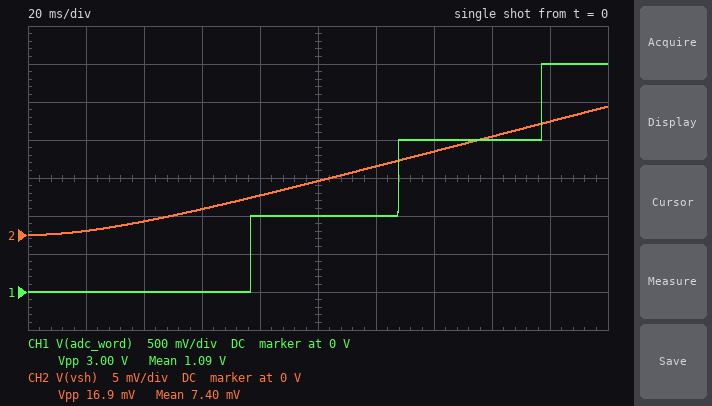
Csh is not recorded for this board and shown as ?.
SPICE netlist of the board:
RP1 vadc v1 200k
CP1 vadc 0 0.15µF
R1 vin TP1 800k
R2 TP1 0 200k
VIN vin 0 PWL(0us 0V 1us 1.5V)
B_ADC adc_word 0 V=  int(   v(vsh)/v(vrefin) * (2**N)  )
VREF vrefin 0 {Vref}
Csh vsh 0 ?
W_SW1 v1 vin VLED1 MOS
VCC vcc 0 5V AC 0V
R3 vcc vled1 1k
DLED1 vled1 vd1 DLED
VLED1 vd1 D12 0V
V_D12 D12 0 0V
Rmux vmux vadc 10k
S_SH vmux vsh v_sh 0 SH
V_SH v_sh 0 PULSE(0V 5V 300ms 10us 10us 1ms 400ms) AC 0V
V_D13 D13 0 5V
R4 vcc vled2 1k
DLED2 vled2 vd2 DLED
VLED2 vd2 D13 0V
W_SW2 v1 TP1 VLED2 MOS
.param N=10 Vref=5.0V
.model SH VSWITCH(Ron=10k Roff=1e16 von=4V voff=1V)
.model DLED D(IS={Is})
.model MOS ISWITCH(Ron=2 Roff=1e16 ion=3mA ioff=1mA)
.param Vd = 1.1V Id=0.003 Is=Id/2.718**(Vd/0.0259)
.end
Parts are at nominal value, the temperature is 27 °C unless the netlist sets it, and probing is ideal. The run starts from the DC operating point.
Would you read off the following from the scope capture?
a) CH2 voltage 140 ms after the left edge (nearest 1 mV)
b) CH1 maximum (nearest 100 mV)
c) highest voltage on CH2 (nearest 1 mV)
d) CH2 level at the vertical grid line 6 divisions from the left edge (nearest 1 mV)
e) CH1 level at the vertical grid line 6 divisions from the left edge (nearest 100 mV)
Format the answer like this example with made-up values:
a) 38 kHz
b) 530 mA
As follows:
a) 11 mV
b) 3.0 V
c) 17 mV
d) 9 mV
e) 1.0 V
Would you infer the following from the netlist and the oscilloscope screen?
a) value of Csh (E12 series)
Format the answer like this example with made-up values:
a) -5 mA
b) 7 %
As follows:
a) 15 pF
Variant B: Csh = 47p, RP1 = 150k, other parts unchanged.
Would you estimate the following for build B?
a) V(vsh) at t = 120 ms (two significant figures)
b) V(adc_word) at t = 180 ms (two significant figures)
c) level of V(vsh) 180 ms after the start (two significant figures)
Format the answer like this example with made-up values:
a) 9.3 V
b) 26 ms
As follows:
a) 3.1 mV
b) 1.0 V
c) 5.0 mV
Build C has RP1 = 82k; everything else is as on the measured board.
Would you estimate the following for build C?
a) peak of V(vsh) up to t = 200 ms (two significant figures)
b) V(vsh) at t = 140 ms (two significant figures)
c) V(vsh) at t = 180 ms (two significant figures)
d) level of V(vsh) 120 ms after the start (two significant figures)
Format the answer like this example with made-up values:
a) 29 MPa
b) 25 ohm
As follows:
a) 19 mV
b) 13 mV
c) 17 mV
d) 11 mV
